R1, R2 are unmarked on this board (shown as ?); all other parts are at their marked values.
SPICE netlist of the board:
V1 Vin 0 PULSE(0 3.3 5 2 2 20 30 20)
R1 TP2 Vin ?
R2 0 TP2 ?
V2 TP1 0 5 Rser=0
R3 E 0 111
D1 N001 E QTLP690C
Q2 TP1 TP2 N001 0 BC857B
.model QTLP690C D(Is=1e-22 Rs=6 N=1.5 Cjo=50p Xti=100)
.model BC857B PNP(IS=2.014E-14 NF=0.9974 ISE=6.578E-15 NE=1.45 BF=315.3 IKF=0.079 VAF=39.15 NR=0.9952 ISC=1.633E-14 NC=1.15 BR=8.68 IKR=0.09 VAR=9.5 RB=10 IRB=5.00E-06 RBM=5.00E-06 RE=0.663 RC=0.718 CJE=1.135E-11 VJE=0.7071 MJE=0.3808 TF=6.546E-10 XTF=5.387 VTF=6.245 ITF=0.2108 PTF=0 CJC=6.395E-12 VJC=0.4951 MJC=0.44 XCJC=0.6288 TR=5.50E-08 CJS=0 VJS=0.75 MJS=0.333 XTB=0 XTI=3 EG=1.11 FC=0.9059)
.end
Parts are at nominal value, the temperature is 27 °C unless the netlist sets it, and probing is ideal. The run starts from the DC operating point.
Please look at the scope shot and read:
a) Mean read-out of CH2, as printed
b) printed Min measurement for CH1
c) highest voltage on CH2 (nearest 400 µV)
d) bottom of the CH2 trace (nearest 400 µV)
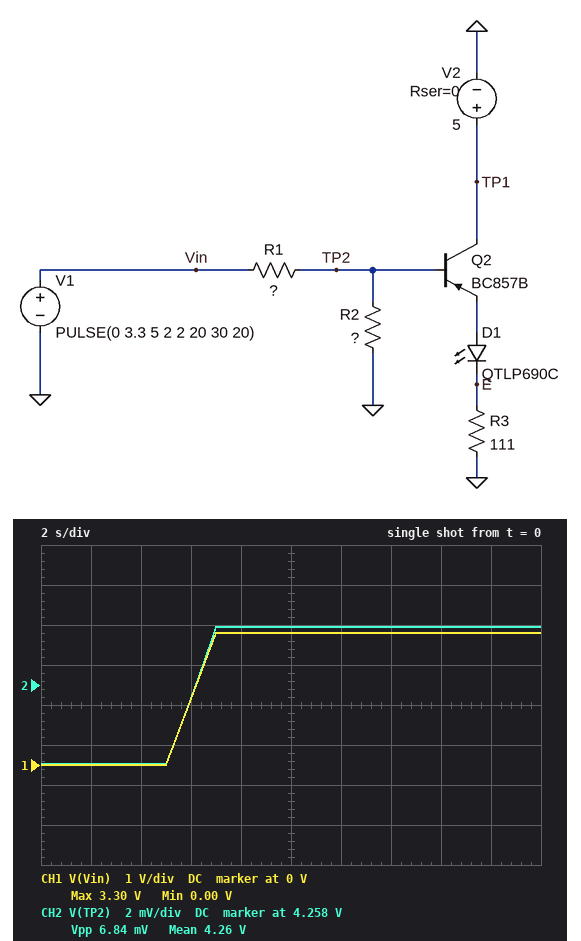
4.26 V
0.00 V
4.2608 V
4.2540 V
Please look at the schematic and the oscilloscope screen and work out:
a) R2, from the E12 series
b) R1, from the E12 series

1.2 kΩ
4.7 kΩ
